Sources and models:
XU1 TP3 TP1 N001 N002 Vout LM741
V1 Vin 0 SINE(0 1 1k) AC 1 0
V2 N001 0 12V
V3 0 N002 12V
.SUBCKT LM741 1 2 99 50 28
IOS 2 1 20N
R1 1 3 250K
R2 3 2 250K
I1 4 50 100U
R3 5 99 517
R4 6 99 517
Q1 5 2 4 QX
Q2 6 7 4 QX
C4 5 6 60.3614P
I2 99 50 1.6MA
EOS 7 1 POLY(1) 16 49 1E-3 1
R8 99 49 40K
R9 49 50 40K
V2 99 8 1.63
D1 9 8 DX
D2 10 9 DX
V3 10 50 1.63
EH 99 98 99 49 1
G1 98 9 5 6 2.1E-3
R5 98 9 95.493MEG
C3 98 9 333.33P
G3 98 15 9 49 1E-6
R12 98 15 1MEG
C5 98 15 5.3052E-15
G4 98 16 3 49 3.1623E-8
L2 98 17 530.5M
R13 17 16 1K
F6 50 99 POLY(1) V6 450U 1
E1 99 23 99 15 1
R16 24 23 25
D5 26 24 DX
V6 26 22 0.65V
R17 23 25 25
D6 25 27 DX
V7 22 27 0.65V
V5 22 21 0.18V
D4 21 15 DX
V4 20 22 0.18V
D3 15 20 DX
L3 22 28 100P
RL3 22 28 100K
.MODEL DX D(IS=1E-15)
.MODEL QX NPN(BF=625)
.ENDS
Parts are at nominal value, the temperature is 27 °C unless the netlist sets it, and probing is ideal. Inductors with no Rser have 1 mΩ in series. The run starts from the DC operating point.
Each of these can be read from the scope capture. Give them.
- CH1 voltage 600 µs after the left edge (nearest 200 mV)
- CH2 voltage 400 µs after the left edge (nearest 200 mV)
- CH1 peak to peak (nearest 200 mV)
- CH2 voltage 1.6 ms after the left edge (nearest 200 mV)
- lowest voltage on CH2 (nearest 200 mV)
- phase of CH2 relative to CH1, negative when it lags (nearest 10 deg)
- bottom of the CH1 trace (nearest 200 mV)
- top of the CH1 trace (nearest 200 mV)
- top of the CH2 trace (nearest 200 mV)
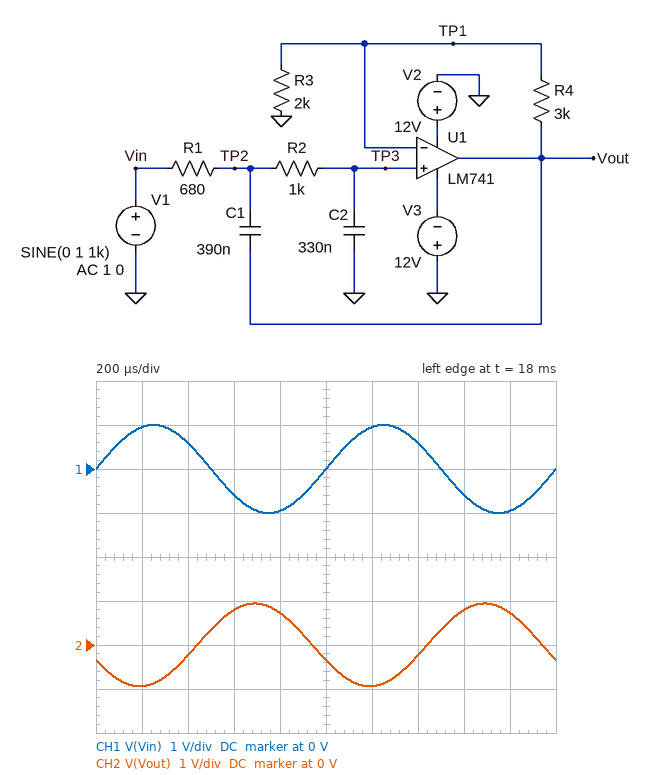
-600 mV
-200 mV
2.0 V
800 mV
-1.0 V
-160 deg
-1.0 V
1.0 V
1.0 V
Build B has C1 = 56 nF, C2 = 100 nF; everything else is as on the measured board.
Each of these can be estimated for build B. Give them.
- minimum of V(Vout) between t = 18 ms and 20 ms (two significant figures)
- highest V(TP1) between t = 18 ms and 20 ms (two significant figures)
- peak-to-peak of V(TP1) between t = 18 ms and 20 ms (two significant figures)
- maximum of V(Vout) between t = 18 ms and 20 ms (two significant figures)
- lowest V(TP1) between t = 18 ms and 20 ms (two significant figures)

-2.3 V
910 mV
1.8 V
2.3 V
-910 mV
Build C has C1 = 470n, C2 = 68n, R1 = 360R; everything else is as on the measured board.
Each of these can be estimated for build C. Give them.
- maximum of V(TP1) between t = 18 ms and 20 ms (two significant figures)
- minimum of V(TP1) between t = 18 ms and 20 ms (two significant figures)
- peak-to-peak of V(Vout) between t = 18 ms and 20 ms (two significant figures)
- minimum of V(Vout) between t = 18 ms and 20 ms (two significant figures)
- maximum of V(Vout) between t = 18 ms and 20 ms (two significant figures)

4.3 V
-4.3 V
21 V
-11 V
11 V
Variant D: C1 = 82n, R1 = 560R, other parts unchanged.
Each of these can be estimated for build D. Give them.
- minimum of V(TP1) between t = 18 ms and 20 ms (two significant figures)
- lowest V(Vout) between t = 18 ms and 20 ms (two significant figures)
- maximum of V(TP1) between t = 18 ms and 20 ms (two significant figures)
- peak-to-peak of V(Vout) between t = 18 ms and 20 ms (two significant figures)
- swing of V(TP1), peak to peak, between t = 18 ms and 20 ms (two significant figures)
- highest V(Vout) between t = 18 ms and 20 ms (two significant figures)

-350 mV
-880 mV
350 mV
1.8 V
710 mV
890 mV
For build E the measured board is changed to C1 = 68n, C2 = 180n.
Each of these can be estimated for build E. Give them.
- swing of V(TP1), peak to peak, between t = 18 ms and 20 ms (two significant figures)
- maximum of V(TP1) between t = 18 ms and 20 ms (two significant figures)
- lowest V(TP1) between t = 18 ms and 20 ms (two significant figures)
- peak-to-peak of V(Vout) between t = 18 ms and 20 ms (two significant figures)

1.2 V
620 mV
-620 mV
3.1 V
